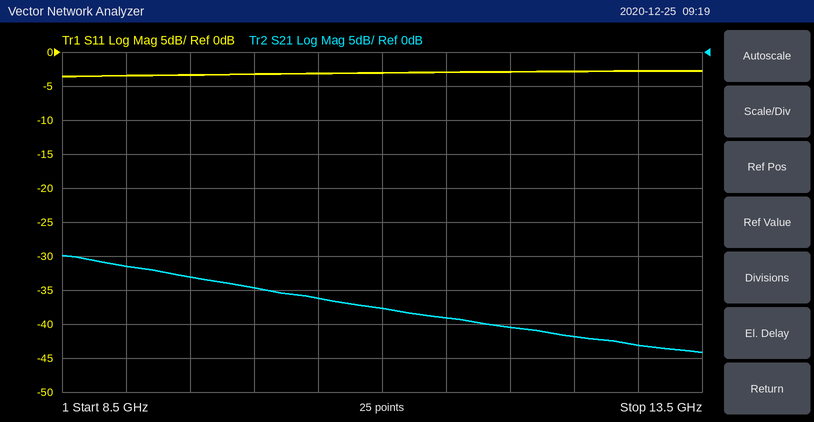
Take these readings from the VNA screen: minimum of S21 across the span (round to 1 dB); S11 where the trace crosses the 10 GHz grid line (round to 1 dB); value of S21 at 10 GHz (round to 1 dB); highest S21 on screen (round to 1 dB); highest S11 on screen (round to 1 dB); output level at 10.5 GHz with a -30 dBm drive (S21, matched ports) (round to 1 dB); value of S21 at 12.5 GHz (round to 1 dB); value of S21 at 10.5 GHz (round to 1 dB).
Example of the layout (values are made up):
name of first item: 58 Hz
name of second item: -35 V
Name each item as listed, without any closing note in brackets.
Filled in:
minimum of S21 across the span: -44 dB
S11 where the trace crosses the 10 GHz grid line: -3 dB
value of S21 at 10 GHz: -35 dB
highest S21 on screen: -30 dB
highest S11 on screen: -3 dB
output level at 10.5 GHz with a -30 dBm drive (S21, matched ports): -66 dBm
value of S21 at 12.5 GHz: -42 dB
value of S21 at 10.5 GHz: -36 dB
